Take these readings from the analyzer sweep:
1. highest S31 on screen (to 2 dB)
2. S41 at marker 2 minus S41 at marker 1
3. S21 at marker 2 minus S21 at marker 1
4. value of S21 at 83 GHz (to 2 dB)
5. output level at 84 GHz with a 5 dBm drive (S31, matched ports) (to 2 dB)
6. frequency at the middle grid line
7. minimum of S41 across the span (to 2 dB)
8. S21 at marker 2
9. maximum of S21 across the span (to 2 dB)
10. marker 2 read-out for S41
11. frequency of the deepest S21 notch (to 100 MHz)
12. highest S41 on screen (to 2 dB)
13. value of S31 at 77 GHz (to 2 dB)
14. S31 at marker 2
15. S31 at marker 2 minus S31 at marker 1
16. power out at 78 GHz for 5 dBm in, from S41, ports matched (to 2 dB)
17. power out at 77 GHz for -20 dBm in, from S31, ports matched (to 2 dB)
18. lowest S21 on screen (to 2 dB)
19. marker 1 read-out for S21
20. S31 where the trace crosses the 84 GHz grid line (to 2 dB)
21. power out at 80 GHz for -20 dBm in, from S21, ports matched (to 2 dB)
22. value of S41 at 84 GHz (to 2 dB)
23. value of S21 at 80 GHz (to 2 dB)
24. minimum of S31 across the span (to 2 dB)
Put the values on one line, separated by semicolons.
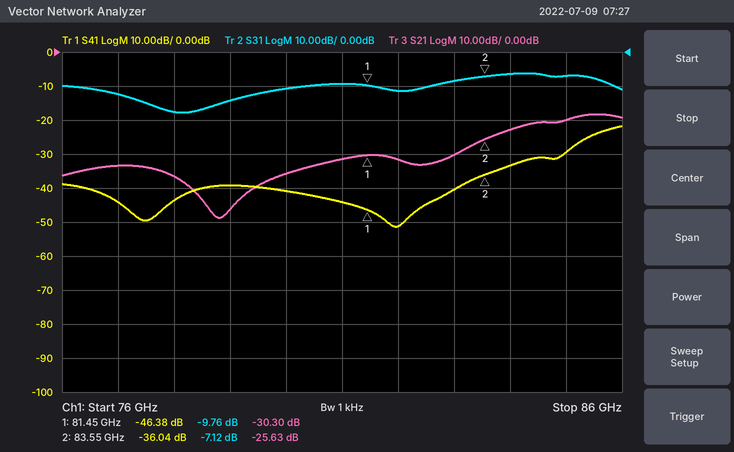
-6 dB; 10.34 dB; 4.67 dB; -30 dB; -2 dBm; 81 GHz; -52 dB; -25.63 dB; -18 dB; -36.04 dB; 78.8 GHz; -22 dB; -12 dB; -7.12 dB; 2.64 dB; -38 dBm; -32 dBm; -48 dB; -30.30 dB; -6 dB; -56 dBm; -34 dB; -36 dB; -18 dB
